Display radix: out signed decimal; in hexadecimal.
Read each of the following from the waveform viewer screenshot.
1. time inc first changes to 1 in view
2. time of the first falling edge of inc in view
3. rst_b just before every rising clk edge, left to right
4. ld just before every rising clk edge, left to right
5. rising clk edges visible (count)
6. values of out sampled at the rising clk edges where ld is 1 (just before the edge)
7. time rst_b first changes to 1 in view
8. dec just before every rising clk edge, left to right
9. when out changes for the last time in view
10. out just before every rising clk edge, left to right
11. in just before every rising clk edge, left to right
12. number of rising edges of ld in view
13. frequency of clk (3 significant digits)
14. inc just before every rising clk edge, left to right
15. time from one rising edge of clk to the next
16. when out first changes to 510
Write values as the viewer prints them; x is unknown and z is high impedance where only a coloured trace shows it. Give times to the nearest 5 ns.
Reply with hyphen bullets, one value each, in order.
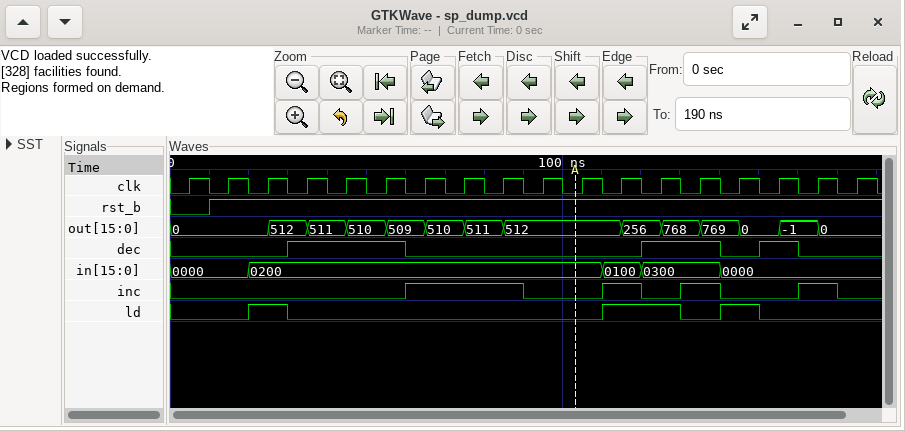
- 60 ns
- 90 ns
- 0 1 1 1 1 1 1 1 1 1 1 1 1 1 1 1 1 1
- 0 0 1 0 0 0 0 0 0 0 0 1 1 0 1 0 0 0
- 18
- 0, 512, 256, 769
- 10 ns
- 0 0 0 1 1 1 0 0 0 0 0 0 1 1 0 1 0 0
- 165 ns
- 0, 0, 0, 512, 511, 510, 509, 510, 511, 512, 512, 512, 256, 768, 769, 0, -1, 0
- 0000, 0000, 0200, 0200, 0200, 0200, 0200, 0200, 0200, 0200, 0200, 0100, 0300, 0300, 0000, 0000, 0000, 0000
- 3
- 100 MHz
- 0 0 0 0 0 0 1 1 1 0 0 1 0 1 0 0 1 0
- 10 ns
- 45 ns
